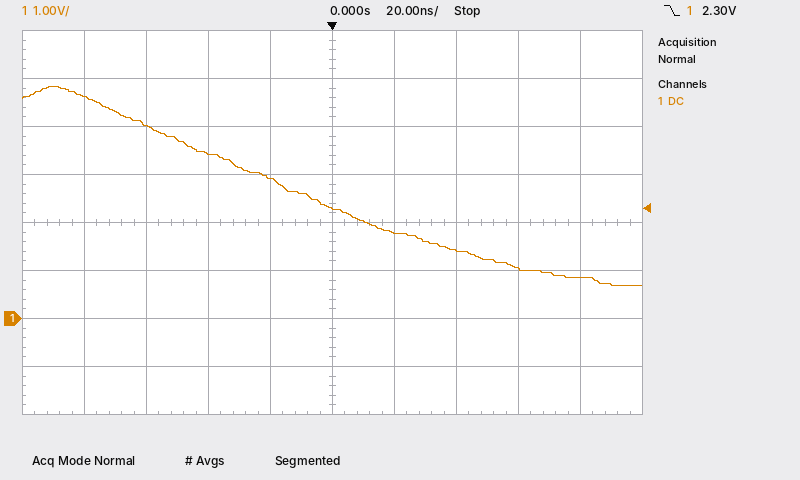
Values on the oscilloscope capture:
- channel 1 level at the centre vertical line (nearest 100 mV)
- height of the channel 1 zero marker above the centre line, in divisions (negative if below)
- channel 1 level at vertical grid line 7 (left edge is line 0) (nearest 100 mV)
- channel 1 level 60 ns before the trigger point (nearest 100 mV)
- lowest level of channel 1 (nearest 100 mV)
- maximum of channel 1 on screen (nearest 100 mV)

2.3 V
-2.0 div
1.4 V
4.0 V
700 mV
4.8 V
